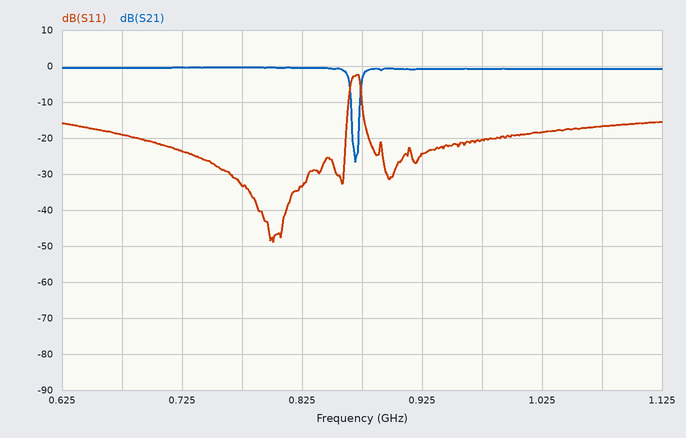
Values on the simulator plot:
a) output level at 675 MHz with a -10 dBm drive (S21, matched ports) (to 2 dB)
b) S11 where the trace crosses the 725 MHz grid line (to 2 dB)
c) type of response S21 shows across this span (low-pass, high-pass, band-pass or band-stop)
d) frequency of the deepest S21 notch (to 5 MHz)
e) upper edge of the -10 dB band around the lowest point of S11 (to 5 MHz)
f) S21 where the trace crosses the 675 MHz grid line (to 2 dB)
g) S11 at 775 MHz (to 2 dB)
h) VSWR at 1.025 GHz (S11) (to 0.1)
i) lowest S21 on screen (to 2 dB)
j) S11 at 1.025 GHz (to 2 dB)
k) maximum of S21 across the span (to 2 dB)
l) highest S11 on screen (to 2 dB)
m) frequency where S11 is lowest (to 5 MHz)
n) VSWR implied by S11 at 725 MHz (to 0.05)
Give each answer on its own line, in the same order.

-10 dBm
-24 dB
band-stop
870 MHz
865 MHz
0 dB
-34 dB
1.3
-26 dB
-18 dB
0 dB
-2 dB
800 MHz
1.15
